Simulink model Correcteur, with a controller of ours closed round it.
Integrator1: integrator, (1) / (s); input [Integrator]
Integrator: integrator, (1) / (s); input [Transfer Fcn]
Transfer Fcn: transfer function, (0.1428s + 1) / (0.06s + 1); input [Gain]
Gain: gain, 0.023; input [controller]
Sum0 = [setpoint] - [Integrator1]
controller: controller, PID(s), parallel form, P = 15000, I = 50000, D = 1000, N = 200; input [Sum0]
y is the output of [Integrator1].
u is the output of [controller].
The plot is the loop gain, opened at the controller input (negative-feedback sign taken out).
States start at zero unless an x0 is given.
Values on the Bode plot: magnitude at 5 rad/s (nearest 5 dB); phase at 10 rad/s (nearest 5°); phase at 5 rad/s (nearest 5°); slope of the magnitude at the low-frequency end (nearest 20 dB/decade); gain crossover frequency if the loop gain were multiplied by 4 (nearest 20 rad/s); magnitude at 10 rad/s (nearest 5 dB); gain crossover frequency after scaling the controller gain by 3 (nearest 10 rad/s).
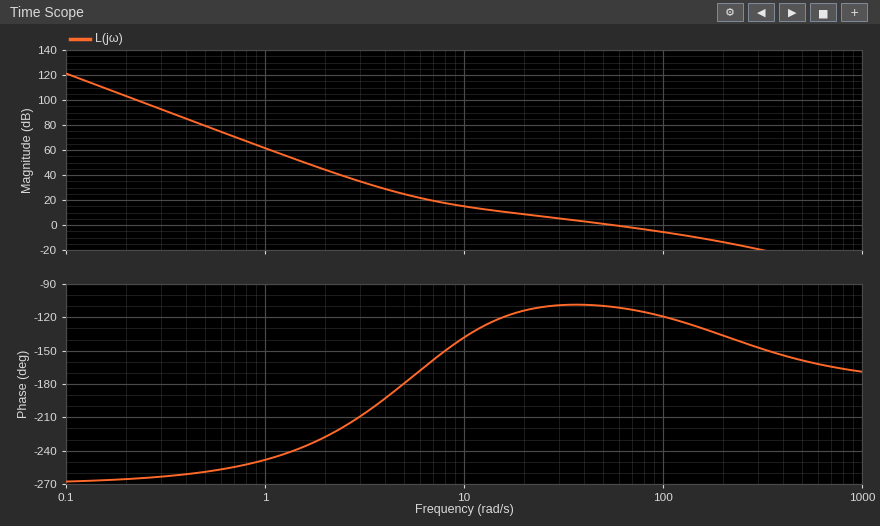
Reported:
25 dB
-140°
-180°
-60 dB/decade
180 rad/s
15 dB
140 rad/s
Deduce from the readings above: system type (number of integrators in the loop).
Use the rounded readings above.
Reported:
3
